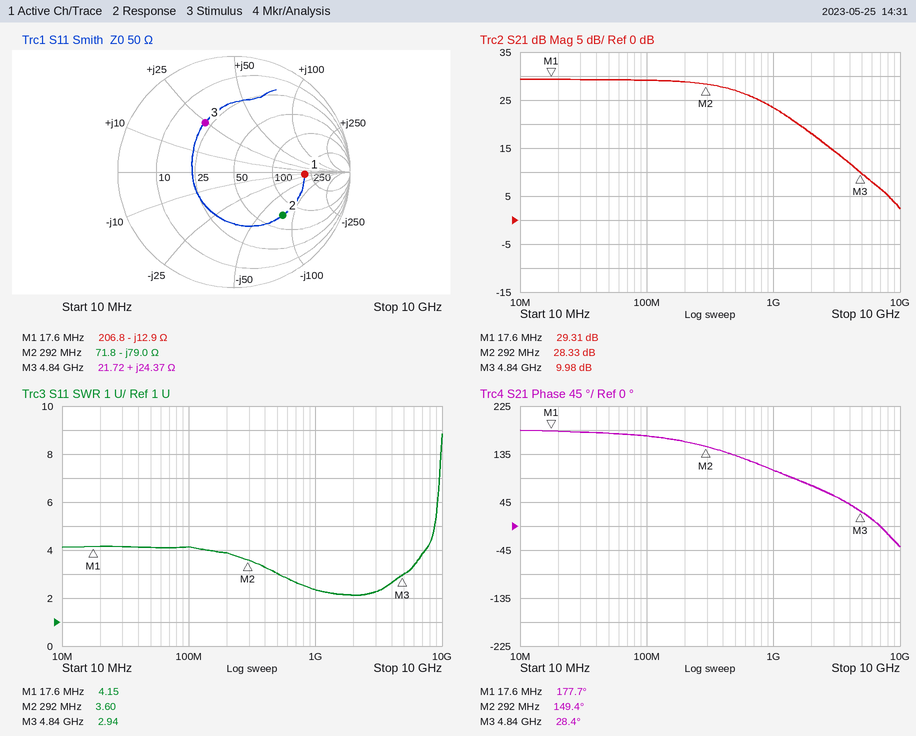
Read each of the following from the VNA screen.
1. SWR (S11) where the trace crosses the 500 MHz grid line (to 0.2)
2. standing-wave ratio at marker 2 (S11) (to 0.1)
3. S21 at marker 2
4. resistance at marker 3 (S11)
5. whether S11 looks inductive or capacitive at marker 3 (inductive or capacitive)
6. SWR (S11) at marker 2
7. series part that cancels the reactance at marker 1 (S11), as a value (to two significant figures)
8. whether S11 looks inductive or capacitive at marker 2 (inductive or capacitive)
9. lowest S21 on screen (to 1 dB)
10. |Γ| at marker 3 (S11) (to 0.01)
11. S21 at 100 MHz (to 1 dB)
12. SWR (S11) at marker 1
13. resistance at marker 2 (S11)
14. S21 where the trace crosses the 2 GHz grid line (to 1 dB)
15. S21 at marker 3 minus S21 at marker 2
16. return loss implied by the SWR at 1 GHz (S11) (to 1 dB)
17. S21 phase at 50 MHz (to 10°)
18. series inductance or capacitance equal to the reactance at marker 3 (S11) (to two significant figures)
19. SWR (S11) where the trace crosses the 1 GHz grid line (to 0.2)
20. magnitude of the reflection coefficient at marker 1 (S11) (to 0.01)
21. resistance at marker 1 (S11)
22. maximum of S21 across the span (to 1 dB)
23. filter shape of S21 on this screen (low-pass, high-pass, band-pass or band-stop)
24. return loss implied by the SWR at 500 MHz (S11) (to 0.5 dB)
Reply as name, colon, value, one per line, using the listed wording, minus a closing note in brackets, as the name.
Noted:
SWR (S11) where the trace crosses the 500 MHz grid line: 3.0
standing-wave ratio at marker 2 (S11): 3.6
S21 at marker 2: 28.33 dB
resistance at marker 3: 21.72 Ω
whether S11 looks inductive or capacitive at marker 3: inductive
SWR (S11) at marker 2: 3.60
series part that cancels the reactance at marker 1 (S11), as a value: 120 nH
whether S11 looks inductive or capacitive at marker 2: capacitive
lowest S21 on screen: 2 dB
|Γ| at marker 3 (S11): 0.49
S21 at 100 MHz: 29 dB
SWR (S11) at marker 1: 4.15
resistance at marker 2: 71.8 Ω
S21 where the trace crosses the 2 GHz grid line: 18 dB
S21 at marker 3 minus S21 at marker 2: -18.35 dB
return loss implied by the SWR at 1 GHz (S11): 8 dB
S21 phase at 50 MHz: 170°
series inductance or capacitance equal to the reactance at marker 3 (S11): 800 pH
SWR (S11) where the trace crosses the 1 GHz grid line: 2.4
magnitude of the reflection coefficient at marker 1 (S11): 0.61
resistance at marker 1: 206.8 Ω
maximum of S21 across the span: 29 dB
filter shape of S21 on this screen: low-pass
return loss implied by the SWR at 500 MHz (S11): 6.0 dB
